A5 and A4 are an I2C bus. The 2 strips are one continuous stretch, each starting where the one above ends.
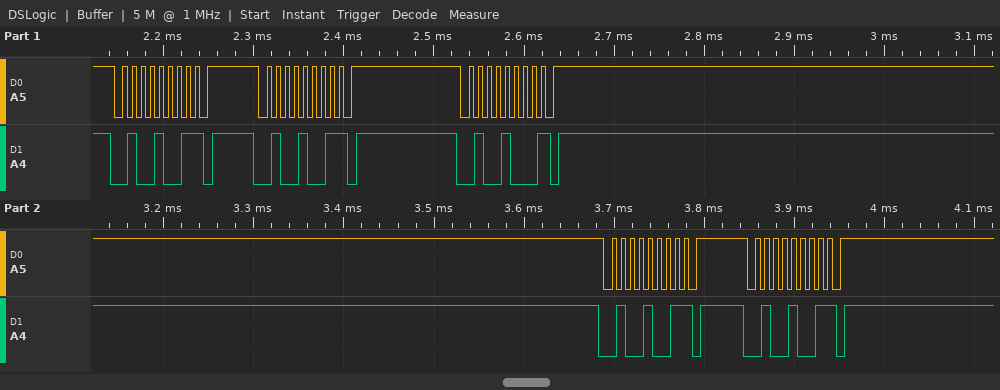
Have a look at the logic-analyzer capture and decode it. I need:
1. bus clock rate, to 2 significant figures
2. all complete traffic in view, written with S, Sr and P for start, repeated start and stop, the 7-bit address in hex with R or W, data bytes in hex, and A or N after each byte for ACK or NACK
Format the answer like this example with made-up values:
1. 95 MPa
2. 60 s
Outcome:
1. 100 kHz
2. S 24R N P S 24R N P S 24W N P S 24R N P S 24R N P
